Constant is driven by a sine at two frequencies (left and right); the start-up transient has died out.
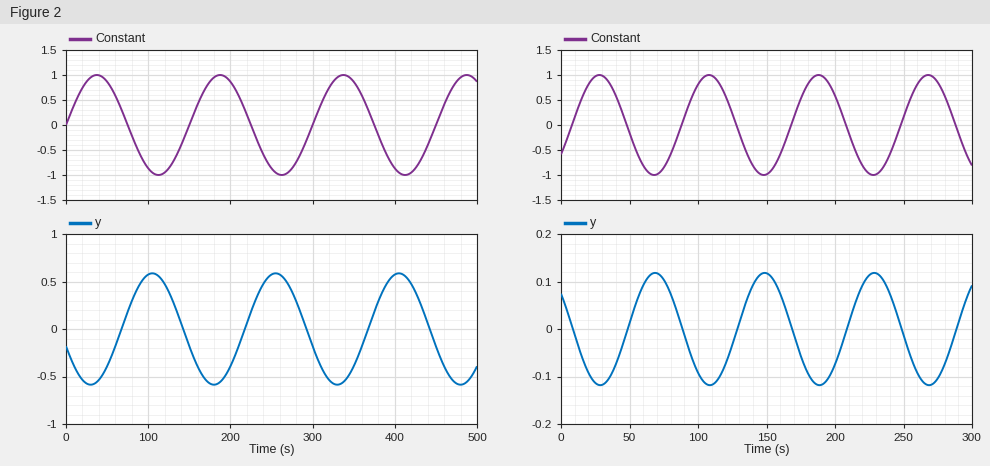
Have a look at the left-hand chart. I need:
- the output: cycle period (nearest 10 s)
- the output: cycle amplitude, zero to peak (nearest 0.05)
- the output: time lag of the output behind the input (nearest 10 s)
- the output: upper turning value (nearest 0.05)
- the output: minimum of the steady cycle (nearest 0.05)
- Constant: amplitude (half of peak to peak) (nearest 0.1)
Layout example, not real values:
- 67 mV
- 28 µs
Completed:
- 150 s
- 0.60
- 70 s
- 0.60
- -0.60
- 1.0
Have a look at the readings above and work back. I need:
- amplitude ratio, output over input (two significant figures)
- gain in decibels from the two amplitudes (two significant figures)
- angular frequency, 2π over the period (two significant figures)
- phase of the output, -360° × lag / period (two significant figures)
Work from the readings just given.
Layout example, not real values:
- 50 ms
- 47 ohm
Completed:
- 0.60
- -4.4 dB
- 0.042 rad/s
- -170°
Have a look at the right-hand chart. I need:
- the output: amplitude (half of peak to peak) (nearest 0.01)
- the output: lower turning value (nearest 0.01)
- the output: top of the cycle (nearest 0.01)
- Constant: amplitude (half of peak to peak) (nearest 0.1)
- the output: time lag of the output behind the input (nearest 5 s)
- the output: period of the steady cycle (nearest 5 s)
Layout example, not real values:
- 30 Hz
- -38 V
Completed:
- 0.12
- -0.12
- 0.12
- 1.0
- 40 s
- 80 s
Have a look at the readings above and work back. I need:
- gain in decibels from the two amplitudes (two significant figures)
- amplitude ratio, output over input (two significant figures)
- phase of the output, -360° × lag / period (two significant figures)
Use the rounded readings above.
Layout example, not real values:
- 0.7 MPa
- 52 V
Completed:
- -18 dB
- 0.12
- -180°
